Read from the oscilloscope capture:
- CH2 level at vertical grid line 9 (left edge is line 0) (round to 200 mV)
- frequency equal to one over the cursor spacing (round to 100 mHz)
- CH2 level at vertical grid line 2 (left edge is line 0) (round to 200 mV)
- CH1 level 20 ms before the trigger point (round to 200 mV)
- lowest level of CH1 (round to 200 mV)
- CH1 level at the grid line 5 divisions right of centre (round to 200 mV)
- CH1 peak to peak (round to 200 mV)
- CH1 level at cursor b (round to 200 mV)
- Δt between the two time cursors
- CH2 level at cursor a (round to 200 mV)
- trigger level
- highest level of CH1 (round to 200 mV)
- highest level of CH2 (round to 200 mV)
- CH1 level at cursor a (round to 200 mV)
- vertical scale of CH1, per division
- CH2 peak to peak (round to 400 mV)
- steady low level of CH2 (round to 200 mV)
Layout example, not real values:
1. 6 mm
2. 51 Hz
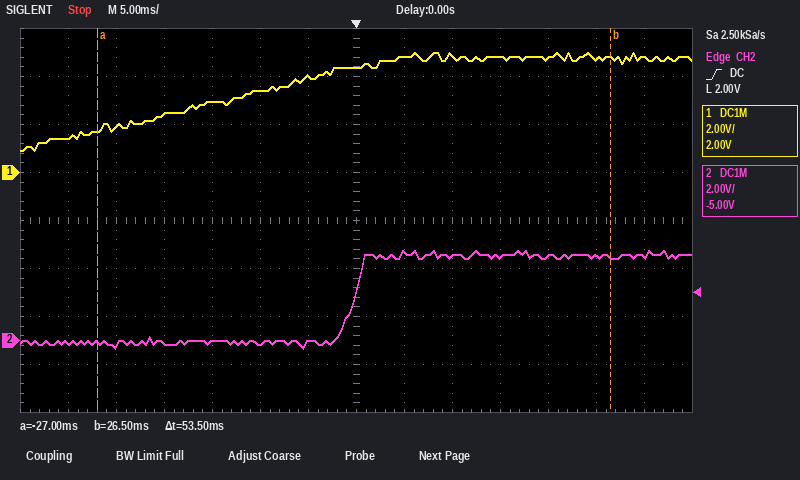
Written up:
1. 3.6 V
2. 18.7 Hz
3. -200 mV
4. 2.4 V
5. 1.0 V
6. 4.8 V
7. 4.0 V
8. 4.8 V
9. 53.5 ms
10. 0.0 V
11. 2.00 V
12. 5.0 V
13. 3.8 V
14. 1.8 V
15. 2 V
16. 4.0 V
17. 0.0 V
